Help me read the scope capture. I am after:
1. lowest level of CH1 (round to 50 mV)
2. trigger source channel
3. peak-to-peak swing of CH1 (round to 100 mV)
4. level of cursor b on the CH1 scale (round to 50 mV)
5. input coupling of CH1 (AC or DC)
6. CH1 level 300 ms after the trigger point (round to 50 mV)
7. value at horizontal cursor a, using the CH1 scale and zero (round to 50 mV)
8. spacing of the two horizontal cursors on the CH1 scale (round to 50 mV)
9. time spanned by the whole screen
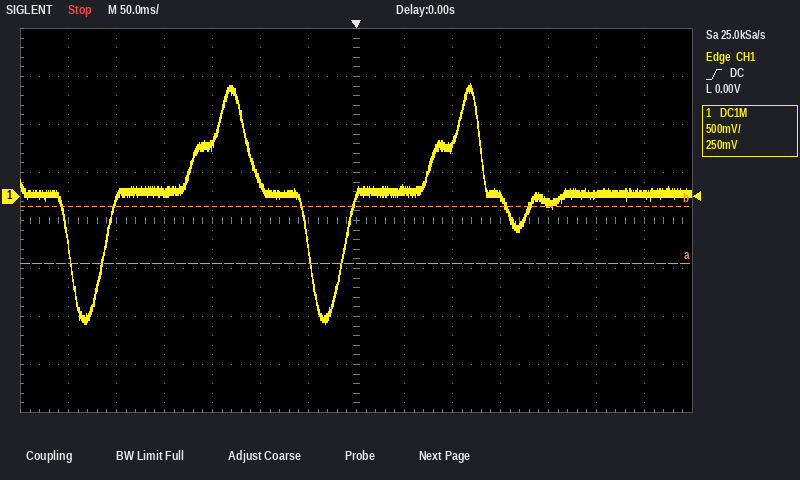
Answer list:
-1.30 V
CH1
2.50 V
-100 mV
DC
50 mV
-700 mV
600 mV
700 ms
